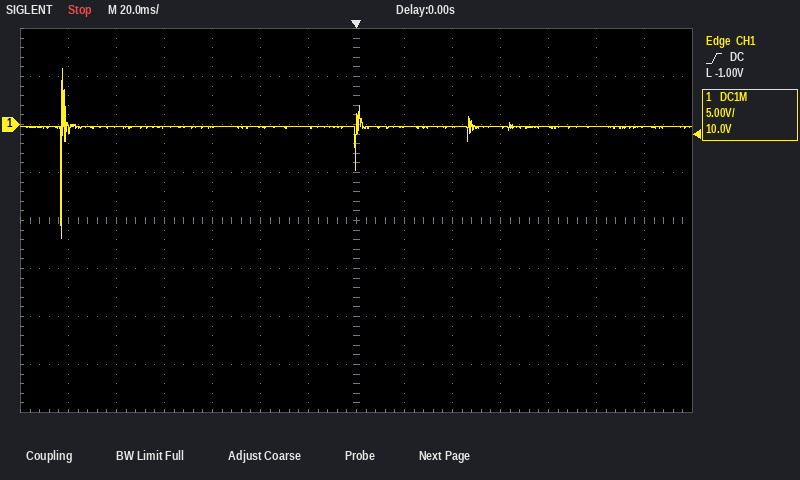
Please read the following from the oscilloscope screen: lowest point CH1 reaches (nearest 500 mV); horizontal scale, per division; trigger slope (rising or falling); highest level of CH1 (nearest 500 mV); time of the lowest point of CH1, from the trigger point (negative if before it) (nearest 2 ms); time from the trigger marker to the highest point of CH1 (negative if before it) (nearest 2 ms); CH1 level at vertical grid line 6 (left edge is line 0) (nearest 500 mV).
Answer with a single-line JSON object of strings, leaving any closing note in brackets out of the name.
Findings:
{"lowest point CH1 reaches": "-12.0 V", "horizontal scale, per division": "20 ms", "trigger slope": "rising", "highest level of CH1": "6.0 V", "time of the lowest point of CH1, from the trigger point (negative if before it)": "-122 ms", "time from the trigger marker to the highest point of CH1 (negative if before it)": "-122 ms", "CH1 level at vertical grid line 6 (left edge is line 0)": "0.0 V"}
